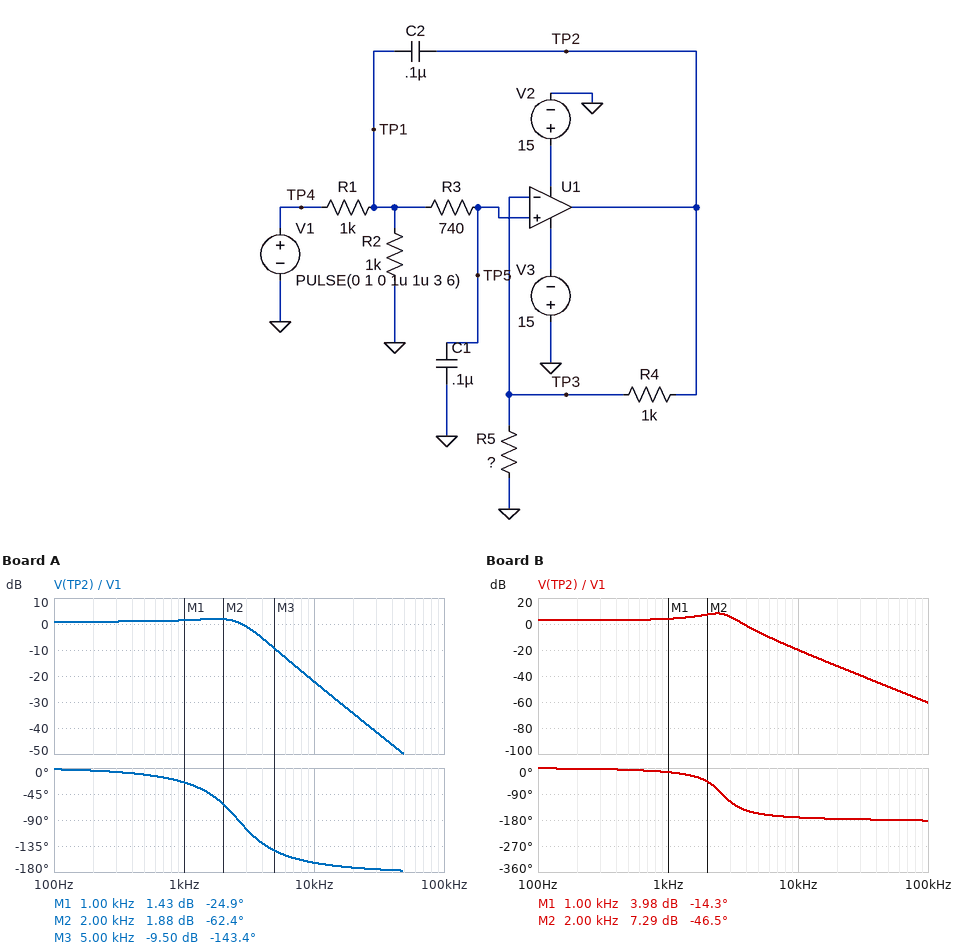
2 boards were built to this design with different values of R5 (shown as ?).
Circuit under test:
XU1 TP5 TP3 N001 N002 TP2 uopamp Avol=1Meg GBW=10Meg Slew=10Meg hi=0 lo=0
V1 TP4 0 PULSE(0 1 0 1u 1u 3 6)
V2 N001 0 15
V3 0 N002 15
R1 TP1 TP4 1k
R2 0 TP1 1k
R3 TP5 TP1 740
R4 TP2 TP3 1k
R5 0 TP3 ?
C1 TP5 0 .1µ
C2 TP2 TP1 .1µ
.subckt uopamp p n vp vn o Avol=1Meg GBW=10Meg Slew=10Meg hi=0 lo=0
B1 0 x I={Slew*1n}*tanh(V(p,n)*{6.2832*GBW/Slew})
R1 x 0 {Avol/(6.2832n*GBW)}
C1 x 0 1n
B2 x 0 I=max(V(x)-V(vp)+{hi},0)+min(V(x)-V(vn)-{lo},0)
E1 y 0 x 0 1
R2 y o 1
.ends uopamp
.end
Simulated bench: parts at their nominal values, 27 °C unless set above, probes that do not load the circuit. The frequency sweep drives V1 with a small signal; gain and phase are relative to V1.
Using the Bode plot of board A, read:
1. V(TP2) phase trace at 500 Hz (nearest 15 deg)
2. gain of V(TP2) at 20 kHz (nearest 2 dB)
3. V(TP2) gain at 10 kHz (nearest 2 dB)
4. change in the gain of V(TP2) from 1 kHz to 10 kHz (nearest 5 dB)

-15 deg
-34 dB
-22 dB
-25 dB
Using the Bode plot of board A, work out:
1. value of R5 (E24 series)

820 Ω
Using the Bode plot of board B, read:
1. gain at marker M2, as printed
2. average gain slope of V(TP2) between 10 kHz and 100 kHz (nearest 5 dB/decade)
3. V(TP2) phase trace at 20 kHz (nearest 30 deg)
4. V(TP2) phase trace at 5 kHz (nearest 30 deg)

7.29 dB
-40 dB/decade
-180 deg
-150 deg
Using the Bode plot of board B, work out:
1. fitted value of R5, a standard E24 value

560 Ω
